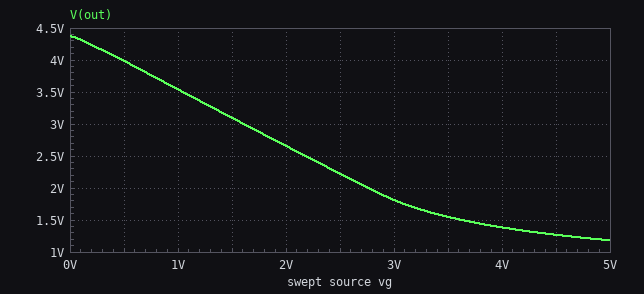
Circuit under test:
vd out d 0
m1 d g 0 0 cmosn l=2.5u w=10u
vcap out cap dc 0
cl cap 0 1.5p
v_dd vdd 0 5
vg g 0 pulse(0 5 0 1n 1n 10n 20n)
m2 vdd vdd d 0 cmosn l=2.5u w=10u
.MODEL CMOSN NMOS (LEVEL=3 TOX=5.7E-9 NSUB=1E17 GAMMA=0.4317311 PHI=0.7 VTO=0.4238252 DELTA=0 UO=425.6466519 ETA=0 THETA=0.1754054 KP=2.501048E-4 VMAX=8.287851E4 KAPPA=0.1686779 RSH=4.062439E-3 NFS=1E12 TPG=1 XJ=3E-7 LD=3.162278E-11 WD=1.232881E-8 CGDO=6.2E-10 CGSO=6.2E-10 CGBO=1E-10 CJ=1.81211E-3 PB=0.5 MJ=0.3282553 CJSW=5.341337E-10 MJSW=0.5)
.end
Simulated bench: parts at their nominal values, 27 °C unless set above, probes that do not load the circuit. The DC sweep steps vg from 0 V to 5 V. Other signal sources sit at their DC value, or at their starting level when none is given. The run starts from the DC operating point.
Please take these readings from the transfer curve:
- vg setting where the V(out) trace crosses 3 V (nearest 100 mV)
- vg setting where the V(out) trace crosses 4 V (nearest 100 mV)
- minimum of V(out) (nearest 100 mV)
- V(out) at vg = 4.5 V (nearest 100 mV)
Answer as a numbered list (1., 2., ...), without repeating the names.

1. 1.6 V
2. 500 mV
3. 1.2 V
4. 1.3 V
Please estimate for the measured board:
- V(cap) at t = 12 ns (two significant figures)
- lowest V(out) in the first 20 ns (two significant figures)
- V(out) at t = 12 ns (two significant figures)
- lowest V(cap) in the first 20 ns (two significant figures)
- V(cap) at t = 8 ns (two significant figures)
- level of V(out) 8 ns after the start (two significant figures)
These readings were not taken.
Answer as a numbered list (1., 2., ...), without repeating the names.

1. 1.7 V
2. 1.2 V
3. 1.7 V
4. 1.2 V
5. 1.2 V
6. 1.2 V
